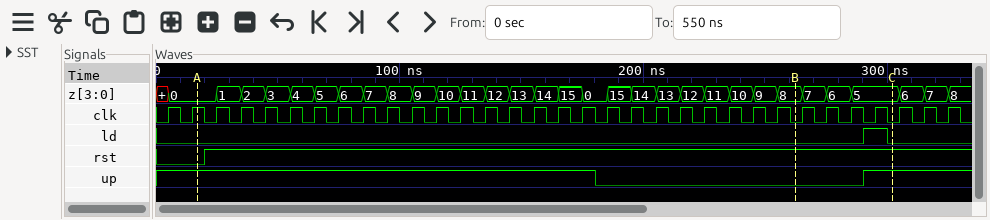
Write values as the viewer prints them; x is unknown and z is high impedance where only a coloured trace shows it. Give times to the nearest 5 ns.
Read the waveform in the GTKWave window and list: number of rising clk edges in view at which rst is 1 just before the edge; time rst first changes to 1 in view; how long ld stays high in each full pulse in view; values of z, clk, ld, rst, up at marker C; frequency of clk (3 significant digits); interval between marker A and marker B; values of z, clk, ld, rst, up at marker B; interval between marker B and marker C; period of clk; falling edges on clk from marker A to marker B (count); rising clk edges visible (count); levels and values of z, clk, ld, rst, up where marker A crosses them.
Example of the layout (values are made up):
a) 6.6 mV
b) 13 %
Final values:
a) 31
b) 20 ns
c) 10 ns
d) z=5, clk=0, ld=0, rst=1, up=1
e) 100 MHz
f) 245 ns
g) z=8, clk=0, ld=0, rst=1, up=0
h) 40 ns
i) 10 ns
j) 25
k) 33
l) z=0, clk=1, ld=0, rst=0, up=1
